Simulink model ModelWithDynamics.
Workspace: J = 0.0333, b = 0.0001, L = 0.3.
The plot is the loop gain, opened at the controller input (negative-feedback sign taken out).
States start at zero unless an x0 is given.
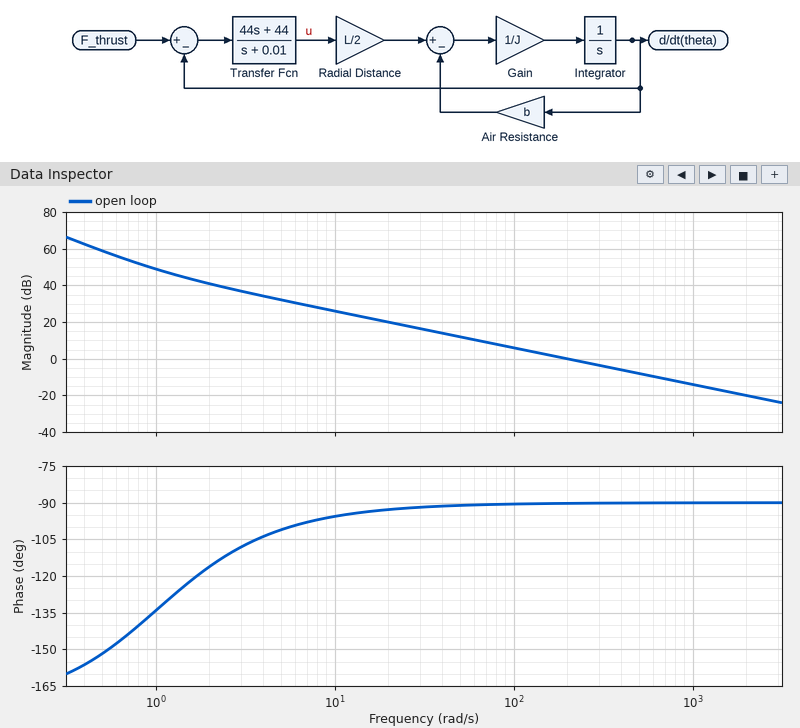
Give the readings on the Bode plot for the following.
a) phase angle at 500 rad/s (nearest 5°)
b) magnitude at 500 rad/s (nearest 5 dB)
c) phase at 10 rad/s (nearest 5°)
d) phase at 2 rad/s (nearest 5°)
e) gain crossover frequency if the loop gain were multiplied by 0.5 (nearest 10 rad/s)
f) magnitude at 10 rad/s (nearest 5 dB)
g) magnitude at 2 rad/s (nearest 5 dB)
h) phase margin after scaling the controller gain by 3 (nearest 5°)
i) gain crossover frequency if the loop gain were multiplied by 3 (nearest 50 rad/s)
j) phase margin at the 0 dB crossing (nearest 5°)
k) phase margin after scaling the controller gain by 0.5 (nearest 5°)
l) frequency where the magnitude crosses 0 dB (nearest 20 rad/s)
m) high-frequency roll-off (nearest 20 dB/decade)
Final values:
-90°
-10 dB
-95°
-115°
100 rad/s
25 dB
40 dB
90°
600 rad/s
90°
90°
200 rad/s
-20 dB/decade
